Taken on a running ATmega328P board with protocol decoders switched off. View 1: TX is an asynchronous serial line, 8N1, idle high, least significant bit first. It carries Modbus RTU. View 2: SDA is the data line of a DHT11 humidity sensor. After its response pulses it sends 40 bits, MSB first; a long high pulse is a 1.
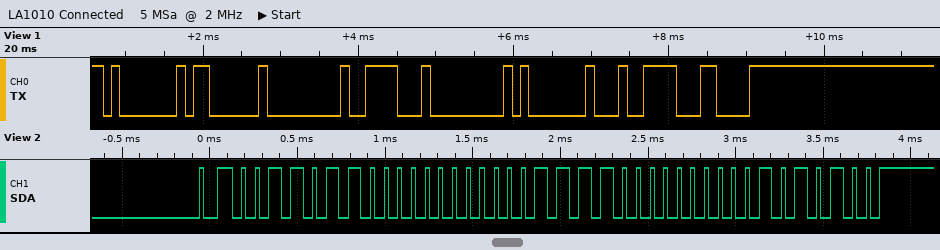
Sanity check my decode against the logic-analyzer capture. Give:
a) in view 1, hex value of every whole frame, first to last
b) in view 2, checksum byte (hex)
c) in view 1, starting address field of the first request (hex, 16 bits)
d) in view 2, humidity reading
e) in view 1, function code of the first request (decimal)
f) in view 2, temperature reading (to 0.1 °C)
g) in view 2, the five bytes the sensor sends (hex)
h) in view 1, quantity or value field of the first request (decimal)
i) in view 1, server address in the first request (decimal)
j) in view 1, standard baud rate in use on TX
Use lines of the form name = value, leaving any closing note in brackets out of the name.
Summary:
in view 1, hex value of every whole frame, first to last = 01 03 00 1E 00 01 E4 0C
in view 2, checksum byte = 0x54
in view 1, starting address field of the first request = 0x001E
in view 2, humidity reading = 54 %
in view 1, function code of the first request = 3
in view 2, temperature reading = 30.0 °C
in view 2, the five bytes the sensor sends = 36 00 1E 00 54
in view 1, quantity or value field of the first request = 1
in view 1, server address in the first request = 1
in view 1, standard baud rate in use on TX = 9600 baud
